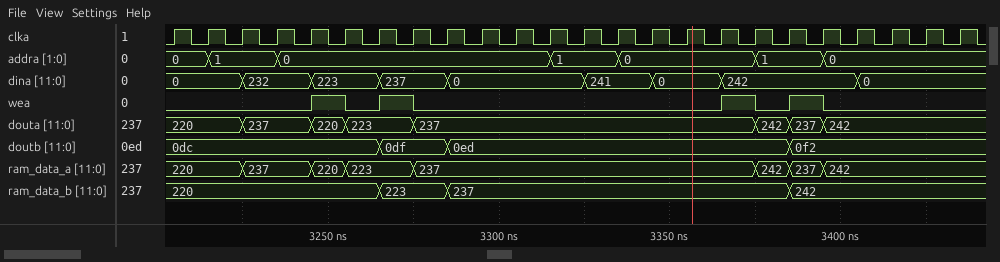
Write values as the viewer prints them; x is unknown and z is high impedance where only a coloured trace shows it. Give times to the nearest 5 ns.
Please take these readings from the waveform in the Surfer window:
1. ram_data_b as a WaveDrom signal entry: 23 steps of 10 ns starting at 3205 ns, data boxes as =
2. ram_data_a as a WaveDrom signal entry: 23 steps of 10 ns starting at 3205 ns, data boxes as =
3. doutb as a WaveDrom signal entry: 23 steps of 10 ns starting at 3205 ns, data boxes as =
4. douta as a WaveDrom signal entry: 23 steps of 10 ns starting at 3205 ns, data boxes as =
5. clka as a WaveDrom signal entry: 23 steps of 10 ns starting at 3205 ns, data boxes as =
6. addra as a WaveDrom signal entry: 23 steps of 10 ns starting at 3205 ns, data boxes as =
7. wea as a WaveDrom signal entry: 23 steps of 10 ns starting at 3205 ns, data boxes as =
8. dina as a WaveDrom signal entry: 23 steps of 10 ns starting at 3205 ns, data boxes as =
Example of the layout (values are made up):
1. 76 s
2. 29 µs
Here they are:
1. {name: 'ram_data_b', wave: '=.....=.=.........=....', data: '220 223 237 242'}
2. {name: 'ram_data_a', wave: '=.=.==.=.........===...', data: '220 237 220 223 237 242 237 242'}
3. {name: 'doutb', wave: '=.....=.=.........=....', data: '0dc 0df 0ed 0f2'}
4. {name: 'douta', wave: '=.=.==.=.........===...', data: '220 237 220 223 237 242 237 242'}
5. {name: 'clka', wave: 'p......................'}
6. {name: 'addra', wave: '==.=.......=.=...=.=...', data: '0 1 0 1 0 1 0'}
7. {name: 'wea', wave: '0...1010........1010...'}
8. {name: 'dina', wave: '=.=.=.=.=...=.=.=...=..', data: '0 232 223 237 0 241 0 242 0'}
